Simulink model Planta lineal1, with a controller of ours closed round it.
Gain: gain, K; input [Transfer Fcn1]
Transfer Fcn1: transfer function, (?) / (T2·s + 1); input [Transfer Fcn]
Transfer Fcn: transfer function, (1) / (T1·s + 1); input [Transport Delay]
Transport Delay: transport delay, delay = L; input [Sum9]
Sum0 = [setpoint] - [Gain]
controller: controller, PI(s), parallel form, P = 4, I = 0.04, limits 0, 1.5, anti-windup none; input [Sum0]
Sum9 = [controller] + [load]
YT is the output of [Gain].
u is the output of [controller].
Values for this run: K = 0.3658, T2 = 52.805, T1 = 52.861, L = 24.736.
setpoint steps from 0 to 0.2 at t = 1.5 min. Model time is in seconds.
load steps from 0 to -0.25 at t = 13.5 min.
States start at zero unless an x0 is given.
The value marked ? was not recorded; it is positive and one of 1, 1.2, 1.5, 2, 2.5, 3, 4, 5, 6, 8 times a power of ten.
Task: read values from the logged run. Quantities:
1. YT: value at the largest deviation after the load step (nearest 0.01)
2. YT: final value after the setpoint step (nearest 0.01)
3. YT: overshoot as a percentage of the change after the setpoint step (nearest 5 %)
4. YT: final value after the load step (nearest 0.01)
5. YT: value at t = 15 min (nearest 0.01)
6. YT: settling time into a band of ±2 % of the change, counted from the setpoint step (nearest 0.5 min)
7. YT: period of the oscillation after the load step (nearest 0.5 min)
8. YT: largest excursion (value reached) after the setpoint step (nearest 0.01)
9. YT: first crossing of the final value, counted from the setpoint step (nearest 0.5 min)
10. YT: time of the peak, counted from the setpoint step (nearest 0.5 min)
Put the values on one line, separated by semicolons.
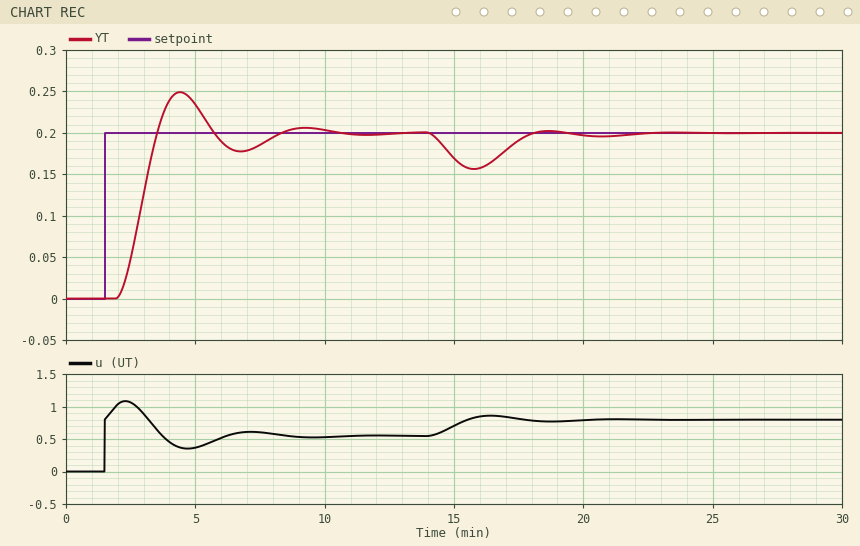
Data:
0.16; 0.20; 25 %; 0.20; 0.17; 8.5 min; 5.0 min; 0.25; 2.0 min; 3.0 min
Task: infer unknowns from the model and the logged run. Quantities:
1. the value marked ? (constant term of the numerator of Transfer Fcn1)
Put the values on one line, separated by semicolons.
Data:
1
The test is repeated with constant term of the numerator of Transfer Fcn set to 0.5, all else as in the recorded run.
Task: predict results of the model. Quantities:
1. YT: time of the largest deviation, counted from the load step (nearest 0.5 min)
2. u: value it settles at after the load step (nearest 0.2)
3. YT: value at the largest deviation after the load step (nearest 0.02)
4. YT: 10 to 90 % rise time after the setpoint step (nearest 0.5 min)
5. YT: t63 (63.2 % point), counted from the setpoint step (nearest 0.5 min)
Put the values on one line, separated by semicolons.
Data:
2.5 min; 1.4; 0.18; 2.5 min; 2.5 min
